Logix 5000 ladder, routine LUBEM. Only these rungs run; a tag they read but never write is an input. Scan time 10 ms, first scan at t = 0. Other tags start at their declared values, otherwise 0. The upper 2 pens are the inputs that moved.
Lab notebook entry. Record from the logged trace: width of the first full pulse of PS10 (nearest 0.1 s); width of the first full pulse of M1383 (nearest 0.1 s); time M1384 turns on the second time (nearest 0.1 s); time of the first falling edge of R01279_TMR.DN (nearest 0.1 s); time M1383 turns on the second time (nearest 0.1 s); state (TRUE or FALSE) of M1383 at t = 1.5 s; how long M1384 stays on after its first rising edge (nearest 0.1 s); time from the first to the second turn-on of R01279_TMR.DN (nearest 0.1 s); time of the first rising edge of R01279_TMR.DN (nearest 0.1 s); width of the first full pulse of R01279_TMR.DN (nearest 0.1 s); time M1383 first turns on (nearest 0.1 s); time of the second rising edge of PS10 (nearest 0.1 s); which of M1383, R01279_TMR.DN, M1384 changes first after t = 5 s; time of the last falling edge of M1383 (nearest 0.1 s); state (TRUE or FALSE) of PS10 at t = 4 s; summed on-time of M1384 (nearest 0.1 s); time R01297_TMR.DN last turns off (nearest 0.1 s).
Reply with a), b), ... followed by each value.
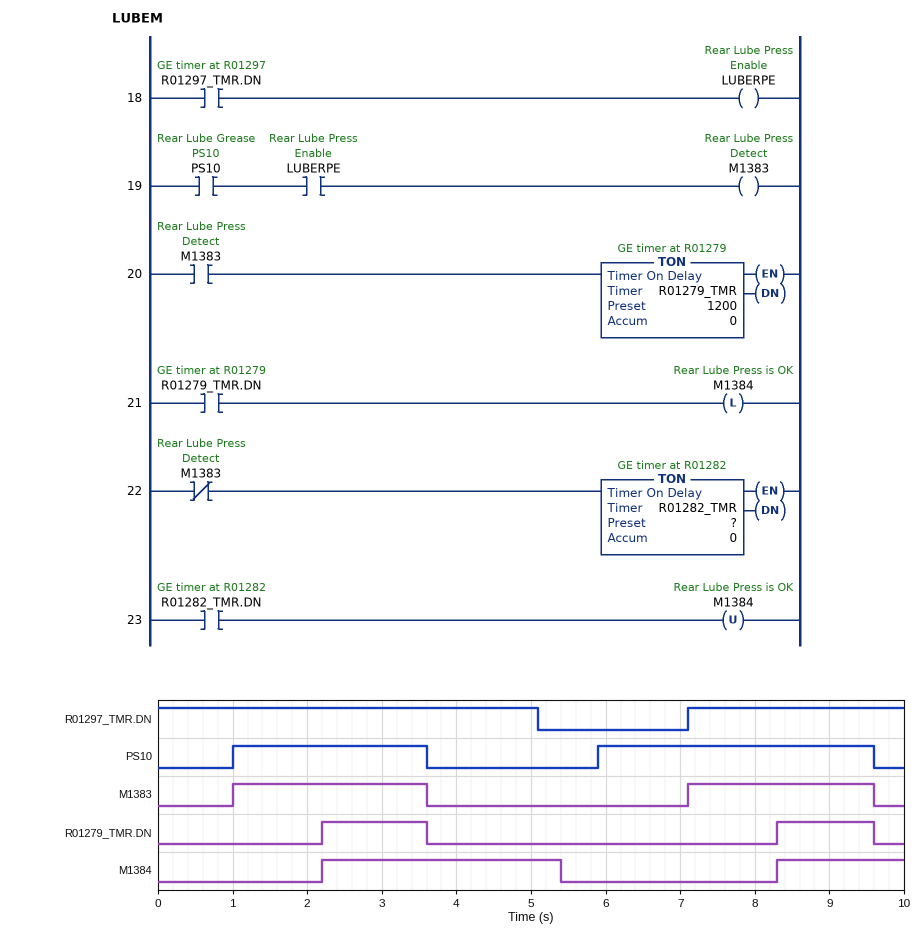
a) 2.6 s
b) 2.6 s
c) 8.3 s
d) 3.6 s
e) 7.1 s
f) TRUE
g) 3.2 s
h) 6.1 s
i) 2.2 s
j) 1.4 s
k) 1.0 s
l) 5.9 s
m) M1384
n) 9.6 s
o) FALSE
p) 4.9 s
q) 5.1 s
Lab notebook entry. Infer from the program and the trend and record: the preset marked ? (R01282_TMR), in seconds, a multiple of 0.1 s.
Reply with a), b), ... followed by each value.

a) 1.8 s
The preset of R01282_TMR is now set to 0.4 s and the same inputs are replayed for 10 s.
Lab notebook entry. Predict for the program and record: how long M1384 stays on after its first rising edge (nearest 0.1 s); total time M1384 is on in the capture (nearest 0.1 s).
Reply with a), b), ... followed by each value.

a) 1.8 s
b) 3.5 s
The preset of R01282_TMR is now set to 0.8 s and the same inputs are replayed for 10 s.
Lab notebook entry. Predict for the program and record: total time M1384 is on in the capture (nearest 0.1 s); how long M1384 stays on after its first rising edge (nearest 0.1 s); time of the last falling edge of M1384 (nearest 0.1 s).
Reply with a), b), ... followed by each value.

a) 3.9 s
b) 2.2 s
c) 4.4 s
